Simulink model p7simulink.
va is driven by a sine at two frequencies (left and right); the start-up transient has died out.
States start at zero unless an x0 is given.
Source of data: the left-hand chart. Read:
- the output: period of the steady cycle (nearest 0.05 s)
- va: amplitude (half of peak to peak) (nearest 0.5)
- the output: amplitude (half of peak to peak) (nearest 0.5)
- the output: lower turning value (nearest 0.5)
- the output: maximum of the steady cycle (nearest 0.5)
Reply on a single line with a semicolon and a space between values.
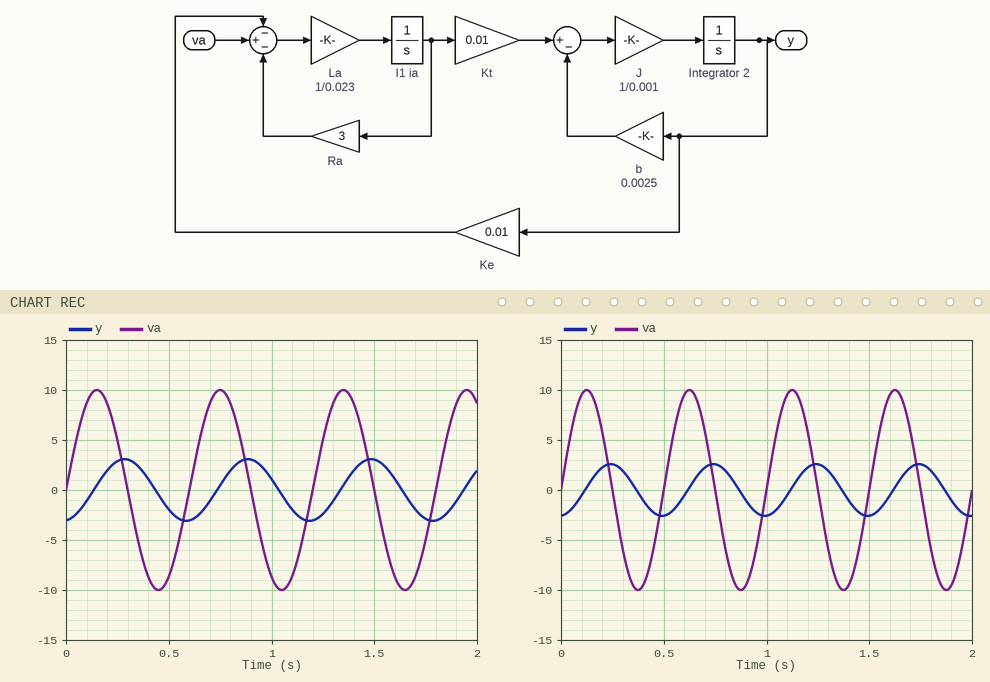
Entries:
0.60 s; 10.0; 3.0; -3.0; 3.0
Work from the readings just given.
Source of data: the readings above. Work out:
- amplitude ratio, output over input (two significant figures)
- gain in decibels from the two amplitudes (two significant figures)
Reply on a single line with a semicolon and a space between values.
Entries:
0.30; -10 dB
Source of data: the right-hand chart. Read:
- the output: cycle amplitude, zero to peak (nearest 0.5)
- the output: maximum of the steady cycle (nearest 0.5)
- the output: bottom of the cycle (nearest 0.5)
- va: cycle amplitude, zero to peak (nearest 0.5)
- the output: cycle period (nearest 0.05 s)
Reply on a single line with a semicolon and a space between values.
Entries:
2.5; 2.5; -2.5; 10.0; 0.50 s
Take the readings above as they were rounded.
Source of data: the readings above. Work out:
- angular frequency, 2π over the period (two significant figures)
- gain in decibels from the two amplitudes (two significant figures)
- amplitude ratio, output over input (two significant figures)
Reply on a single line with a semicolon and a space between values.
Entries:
13 rad/s; -12 dB; 0.25
